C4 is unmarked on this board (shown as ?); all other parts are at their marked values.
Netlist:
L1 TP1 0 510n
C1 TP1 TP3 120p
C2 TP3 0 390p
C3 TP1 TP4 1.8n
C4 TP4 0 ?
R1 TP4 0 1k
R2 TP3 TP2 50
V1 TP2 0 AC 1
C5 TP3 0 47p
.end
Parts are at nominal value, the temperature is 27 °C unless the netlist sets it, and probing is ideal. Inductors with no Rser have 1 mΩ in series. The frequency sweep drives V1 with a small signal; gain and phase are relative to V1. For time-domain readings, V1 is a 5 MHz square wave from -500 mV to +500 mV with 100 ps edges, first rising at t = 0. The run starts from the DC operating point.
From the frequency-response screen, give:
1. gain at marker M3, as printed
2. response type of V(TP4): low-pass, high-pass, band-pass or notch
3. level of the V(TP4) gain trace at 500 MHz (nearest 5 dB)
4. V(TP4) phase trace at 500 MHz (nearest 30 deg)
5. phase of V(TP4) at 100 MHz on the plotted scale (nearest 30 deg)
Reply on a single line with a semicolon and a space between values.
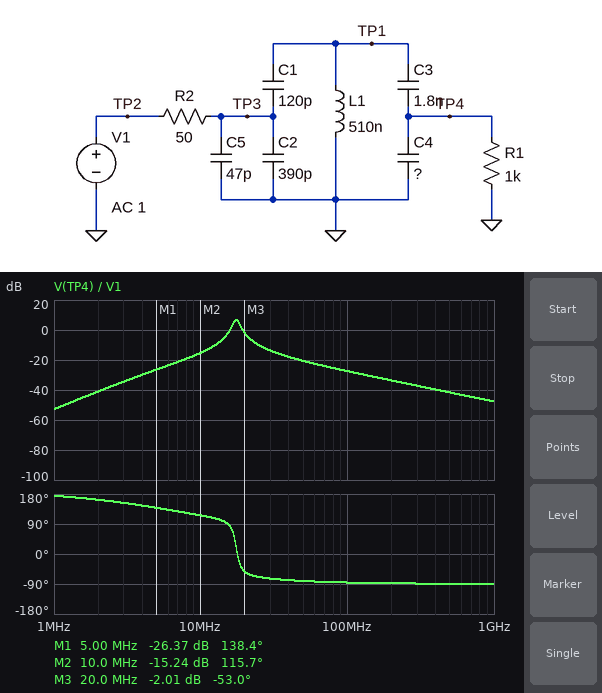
-2.01 dB; band-pass; -40 dB; -90 deg; -90 deg
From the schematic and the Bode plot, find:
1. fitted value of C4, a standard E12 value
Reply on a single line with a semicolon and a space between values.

68 pF
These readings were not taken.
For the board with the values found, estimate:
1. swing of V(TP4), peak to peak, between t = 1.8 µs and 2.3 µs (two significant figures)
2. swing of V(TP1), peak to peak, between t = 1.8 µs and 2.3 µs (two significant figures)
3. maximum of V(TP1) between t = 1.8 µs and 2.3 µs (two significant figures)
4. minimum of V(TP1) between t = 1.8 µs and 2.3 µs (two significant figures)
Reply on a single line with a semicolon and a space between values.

370 mV; 380 mV; 190 mV; -190 mV
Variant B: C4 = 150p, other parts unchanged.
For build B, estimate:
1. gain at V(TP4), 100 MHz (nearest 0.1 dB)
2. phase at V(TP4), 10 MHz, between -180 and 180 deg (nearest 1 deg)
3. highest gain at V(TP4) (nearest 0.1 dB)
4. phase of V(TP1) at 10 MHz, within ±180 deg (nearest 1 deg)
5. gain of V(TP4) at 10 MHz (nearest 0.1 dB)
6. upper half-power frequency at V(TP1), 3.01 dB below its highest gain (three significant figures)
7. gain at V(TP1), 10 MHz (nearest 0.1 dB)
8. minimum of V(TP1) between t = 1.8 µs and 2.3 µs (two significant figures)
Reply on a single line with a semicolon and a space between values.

-31.1 dB; 115 deg; 7.0 dB; 114 deg; -13.5 dB; 15.1 MHz; -12.8 dB; -410 mV
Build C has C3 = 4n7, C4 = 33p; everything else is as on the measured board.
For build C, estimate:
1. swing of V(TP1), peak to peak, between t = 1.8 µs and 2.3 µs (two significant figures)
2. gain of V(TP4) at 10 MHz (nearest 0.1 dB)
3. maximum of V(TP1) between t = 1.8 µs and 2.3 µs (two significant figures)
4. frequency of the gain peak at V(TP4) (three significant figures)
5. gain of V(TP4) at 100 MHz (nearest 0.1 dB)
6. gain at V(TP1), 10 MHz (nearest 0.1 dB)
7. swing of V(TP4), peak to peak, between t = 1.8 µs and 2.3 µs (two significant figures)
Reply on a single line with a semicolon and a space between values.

330 mV; -15.8 dB; 160 mV; 19.6 MHz; -25.1 dB; -15.7 dB; 320 mV
